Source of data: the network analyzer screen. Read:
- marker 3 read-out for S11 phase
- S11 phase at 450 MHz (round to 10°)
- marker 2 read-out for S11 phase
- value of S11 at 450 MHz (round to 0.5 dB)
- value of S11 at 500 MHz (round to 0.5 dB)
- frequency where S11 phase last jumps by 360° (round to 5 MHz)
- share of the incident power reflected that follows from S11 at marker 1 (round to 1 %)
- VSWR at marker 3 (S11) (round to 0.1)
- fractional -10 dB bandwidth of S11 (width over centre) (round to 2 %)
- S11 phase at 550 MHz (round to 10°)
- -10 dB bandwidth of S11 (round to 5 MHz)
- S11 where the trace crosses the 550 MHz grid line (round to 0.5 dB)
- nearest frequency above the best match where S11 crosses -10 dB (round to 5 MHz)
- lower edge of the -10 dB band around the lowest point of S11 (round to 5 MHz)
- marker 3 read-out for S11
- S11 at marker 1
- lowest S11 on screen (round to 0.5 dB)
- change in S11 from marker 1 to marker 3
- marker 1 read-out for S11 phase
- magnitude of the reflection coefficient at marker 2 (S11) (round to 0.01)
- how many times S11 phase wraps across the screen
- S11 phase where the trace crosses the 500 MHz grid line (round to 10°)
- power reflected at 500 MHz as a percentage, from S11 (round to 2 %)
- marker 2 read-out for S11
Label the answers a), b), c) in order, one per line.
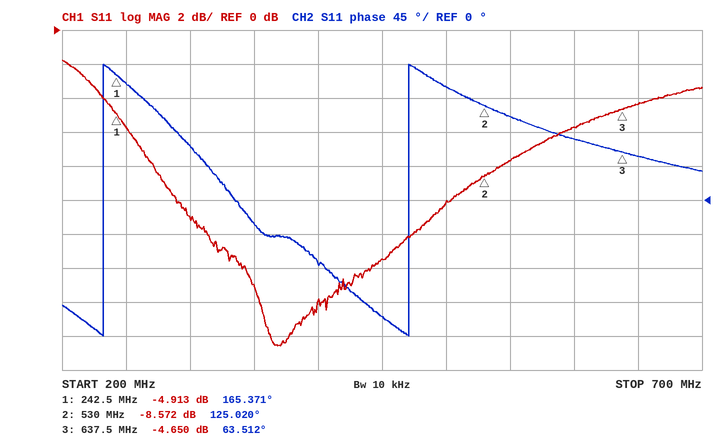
a) 63.512°
b) -150°
c) 125.020°
d) -13.5 dB
e) -10.0 dB
f) 470 MHz
g) 32 %
h) 3.8
i) 54 %
j) 110°
k) 215 MHz
l) -7.5 dB
m) 505 MHz
n) 290 MHz
o) -4.650 dB
p) -4.913 dB
q) -18.5 dB
r) 0.263 dB
s) 165.371°
t) 0.37
u) 2
v) 150°
w) 10 %
x) -8.572 dB
